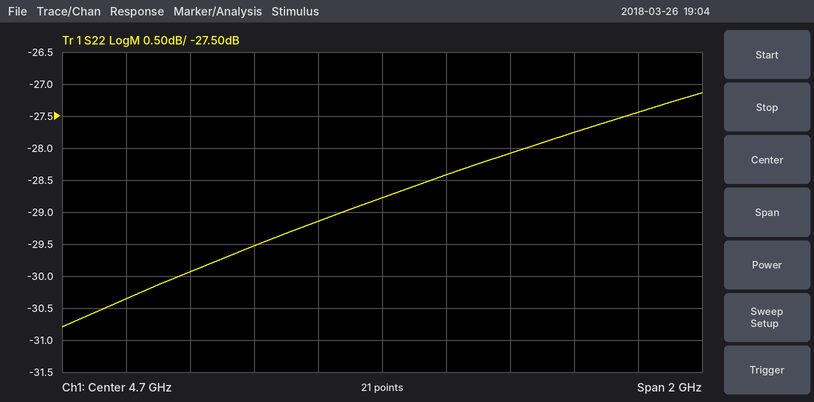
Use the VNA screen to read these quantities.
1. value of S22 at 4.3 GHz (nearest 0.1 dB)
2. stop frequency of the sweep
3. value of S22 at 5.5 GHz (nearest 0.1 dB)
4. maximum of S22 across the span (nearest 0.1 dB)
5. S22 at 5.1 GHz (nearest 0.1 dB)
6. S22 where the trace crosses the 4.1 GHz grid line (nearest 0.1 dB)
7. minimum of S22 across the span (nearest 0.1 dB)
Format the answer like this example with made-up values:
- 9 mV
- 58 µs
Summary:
- -29.5 dB
- 5.7 GHz
- -27.4 dB
- -27.1 dB
- -28.1 dB
- -29.9 dB
- -30.8 dB
